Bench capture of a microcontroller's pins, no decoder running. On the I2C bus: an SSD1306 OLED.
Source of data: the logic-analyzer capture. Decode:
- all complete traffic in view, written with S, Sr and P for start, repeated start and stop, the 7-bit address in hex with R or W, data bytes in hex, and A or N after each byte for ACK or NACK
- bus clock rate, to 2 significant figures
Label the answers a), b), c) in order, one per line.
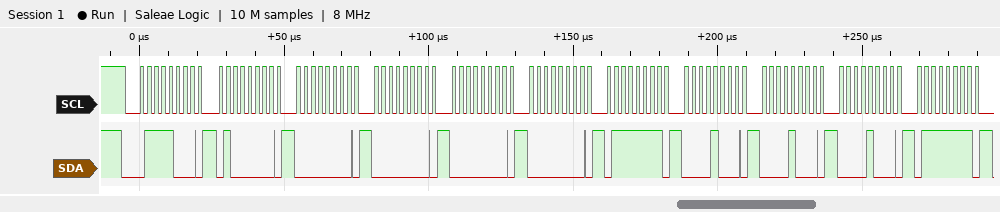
a) S 3CW A 40 A 00 A 00 A 00 A 00 A 7F A 08 A 08 A 08 A 7F A
b) 400 kHz
